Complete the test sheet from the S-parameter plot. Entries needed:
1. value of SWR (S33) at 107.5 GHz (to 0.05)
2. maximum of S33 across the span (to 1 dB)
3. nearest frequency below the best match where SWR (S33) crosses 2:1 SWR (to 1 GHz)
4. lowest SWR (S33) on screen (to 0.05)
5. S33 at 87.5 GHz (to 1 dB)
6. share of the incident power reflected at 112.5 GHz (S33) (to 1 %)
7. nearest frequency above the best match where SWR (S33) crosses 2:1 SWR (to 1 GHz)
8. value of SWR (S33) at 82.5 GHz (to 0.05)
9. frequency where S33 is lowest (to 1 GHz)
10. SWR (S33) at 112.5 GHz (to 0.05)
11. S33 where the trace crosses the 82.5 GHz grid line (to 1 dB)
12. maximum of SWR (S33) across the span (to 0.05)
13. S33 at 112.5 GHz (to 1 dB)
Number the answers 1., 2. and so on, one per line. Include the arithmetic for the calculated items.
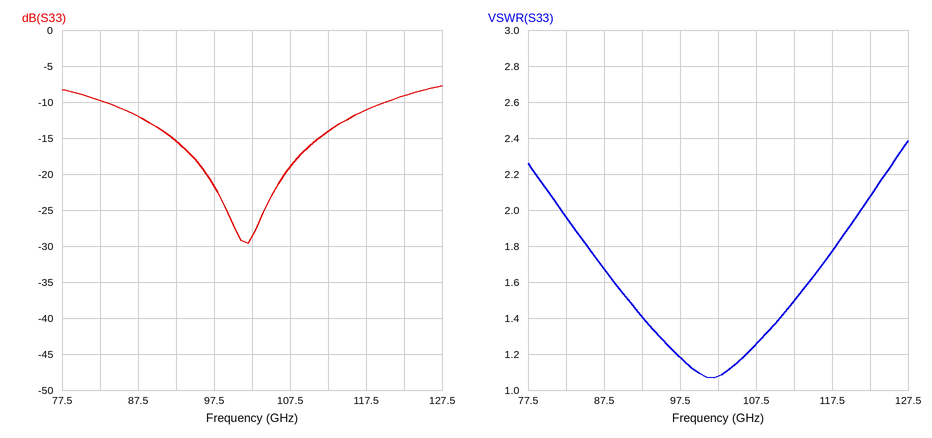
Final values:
1. 1.25
2. -8 dB
3. 82 GHz
4. 1.05
5. -12 dB
6. 10^(-14/10) ≈ 4 %
7. 121 GHz
8. 1.95
9. 102 GHz
10. 1.50
11. -10 dB
12. 2.40
13. -14 dB
